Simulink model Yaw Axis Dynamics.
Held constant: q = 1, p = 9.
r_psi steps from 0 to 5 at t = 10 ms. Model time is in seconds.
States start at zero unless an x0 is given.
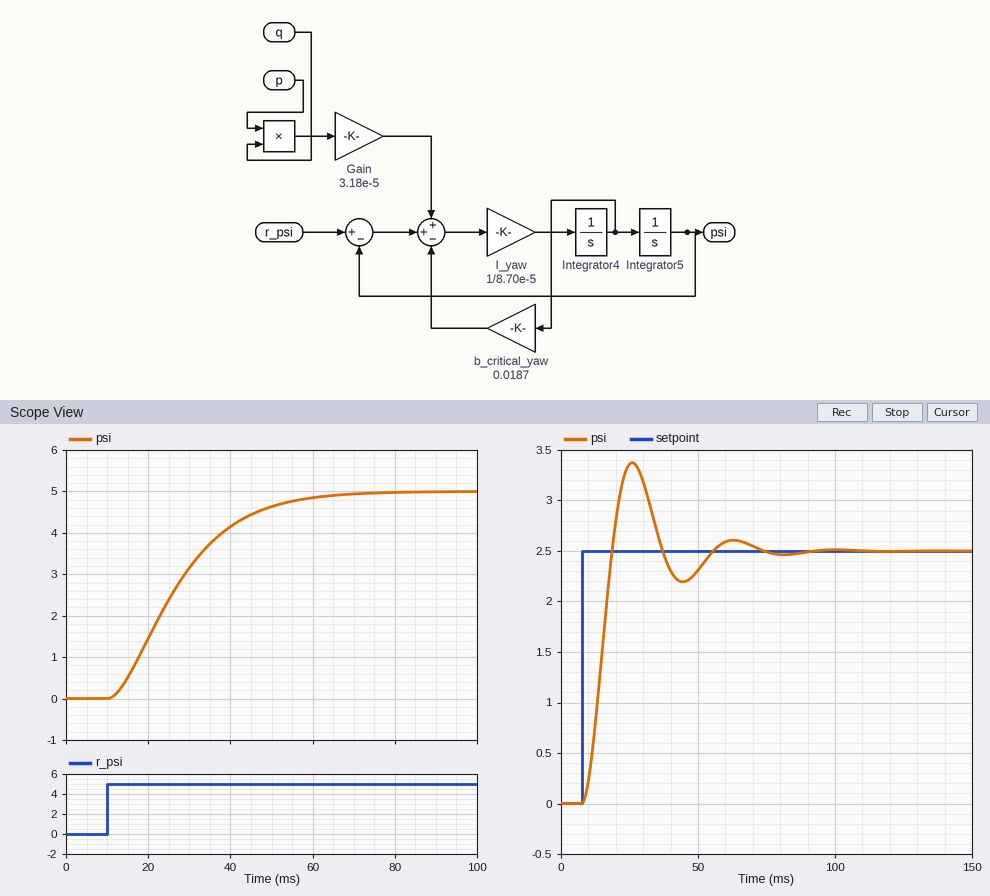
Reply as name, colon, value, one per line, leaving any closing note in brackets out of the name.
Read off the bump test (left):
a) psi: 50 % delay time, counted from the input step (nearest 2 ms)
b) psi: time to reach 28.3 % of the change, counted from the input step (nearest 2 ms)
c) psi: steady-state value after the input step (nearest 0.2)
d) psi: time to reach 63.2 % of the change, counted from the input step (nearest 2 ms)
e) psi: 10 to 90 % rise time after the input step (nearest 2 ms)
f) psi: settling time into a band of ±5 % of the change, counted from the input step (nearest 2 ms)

psi: 50 % delay time, counted from the input step: 16 ms
psi: time to reach 28.3 % of the change, counted from the input step: 10 ms
psi: steady-state value after the input step: 5.0
psi: time to reach 63.2 % of the change, counted from the input step: 20 ms
psi: 10 to 90 % rise time after the input step: 32 ms
psi: settling time into a band of ±5 % of the change, counted from the input step: 44 ms
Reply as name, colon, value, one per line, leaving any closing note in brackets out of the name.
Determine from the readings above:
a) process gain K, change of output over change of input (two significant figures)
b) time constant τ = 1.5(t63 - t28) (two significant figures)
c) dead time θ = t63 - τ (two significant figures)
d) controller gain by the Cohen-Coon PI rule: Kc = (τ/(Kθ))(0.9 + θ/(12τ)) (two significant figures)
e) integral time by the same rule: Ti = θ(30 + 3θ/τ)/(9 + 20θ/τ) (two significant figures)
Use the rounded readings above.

process gain K, change of output over change of input: 1.0
time constant τ = 1.5(t63 - t28): 15 ms
dead time θ = t63 - τ: 5.0 ms
controller gain by the Cohen-Coon PI rule: Kc = (τ/(Kθ))(0.9 + θ/(12τ)): 2.8
integral time by the same rule: Ti = θ(30 + 3θ/τ)/(9 + 20θ/τ): 9.9 ms
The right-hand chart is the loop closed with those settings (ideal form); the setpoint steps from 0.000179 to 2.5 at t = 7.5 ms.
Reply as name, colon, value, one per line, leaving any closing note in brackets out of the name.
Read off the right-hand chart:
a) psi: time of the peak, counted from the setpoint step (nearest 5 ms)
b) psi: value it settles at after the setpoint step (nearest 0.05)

psi: time of the peak, counted from the setpoint step: 20 ms
psi: value it settles at after the setpoint step: 2.50
